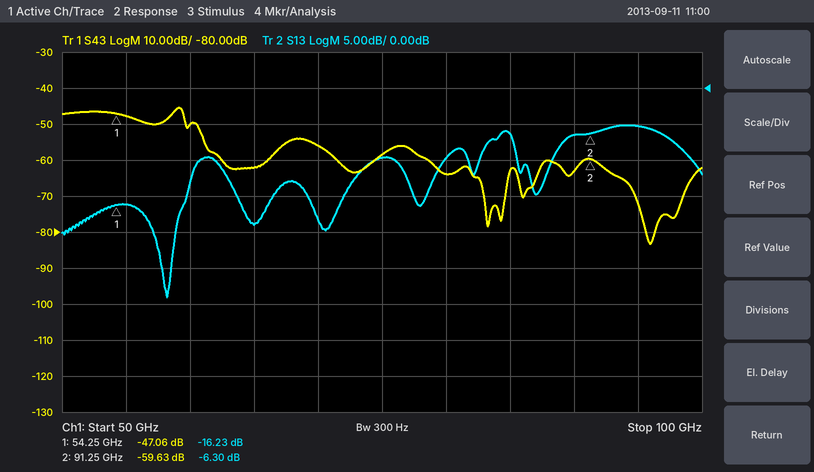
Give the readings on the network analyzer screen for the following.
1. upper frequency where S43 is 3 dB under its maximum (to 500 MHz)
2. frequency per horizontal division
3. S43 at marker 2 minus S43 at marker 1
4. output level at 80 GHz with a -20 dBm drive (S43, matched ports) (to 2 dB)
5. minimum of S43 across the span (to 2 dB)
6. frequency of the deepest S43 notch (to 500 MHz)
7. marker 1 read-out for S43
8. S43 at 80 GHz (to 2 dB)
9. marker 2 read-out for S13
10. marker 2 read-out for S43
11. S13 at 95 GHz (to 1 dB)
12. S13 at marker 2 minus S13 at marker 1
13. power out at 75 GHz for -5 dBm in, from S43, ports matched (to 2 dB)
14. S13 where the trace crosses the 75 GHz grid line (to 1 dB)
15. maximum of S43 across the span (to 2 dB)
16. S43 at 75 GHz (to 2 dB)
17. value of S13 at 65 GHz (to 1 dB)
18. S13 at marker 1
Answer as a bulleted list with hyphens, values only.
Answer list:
- 59.5 GHz
- 5 GHz
- -12.57 dB
- -84 dBm
- -84 dB
- 96.0 GHz
- -47.06 dB
- -64 dB
- -6.30 dB
- -59.63 dB
- -5 dB
- 9.93 dB
- -64 dBm
- -10 dB
- -46 dB
- -58 dB
- -19 dB
- -16.23 dB
